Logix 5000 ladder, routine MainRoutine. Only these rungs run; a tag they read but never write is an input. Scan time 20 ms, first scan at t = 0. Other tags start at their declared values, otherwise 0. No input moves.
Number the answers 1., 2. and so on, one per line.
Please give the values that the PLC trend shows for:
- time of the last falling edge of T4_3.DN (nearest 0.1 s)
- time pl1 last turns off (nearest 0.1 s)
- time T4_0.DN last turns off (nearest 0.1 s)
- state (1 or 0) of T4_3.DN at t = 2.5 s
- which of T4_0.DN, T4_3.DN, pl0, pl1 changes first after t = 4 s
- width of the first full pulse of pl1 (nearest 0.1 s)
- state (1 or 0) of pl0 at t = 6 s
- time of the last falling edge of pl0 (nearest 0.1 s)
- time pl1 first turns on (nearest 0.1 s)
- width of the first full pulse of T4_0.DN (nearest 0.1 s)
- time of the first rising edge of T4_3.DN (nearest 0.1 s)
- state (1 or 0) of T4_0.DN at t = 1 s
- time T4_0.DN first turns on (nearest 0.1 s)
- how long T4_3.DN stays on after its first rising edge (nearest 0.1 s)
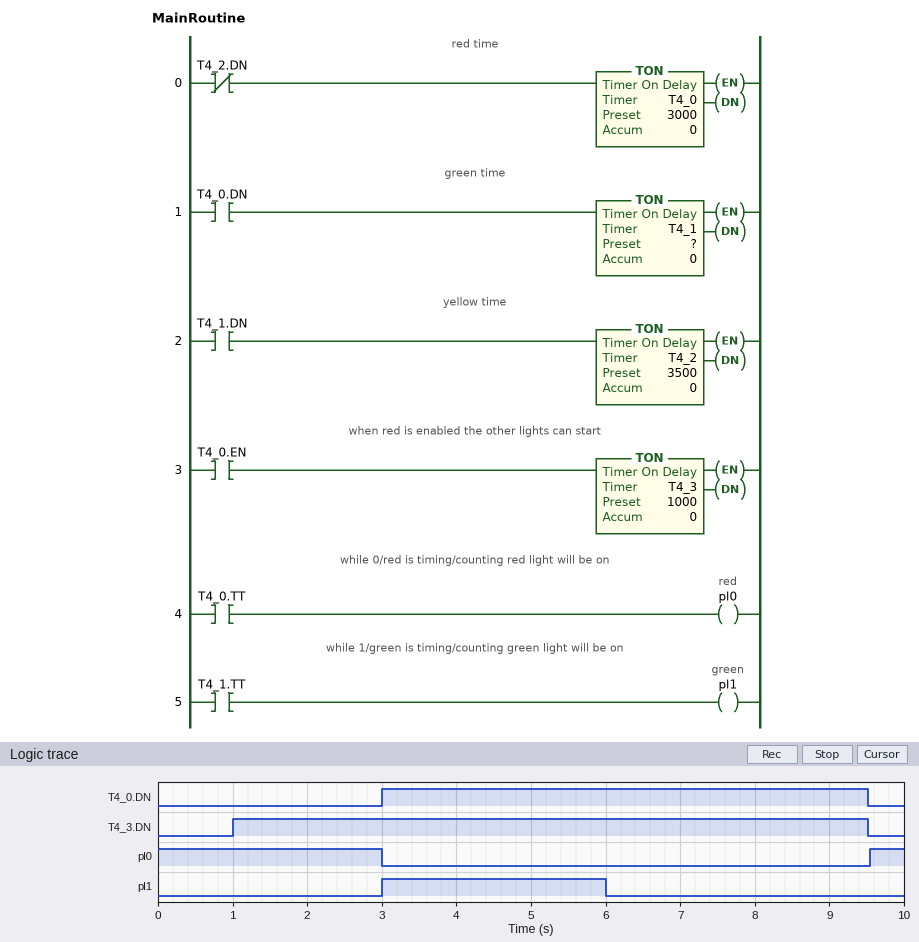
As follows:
1. 9.5 s
2. 6.0 s
3. 9.5 s
4. 1
5. pl1
6. 3.0 s
7. 0
8. 3.0 s
9. 3.0 s
10. 6.5 s
11. 1.0 s
12. 0
13. 3.0 s
14. 8.5 s
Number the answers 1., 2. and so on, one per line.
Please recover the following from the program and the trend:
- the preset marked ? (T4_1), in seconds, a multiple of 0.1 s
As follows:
1. 3.0 s
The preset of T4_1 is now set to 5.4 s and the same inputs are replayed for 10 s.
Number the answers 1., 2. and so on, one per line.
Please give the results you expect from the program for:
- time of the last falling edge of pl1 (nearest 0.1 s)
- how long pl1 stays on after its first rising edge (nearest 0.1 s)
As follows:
1. 8.4 s
2. 5.4 s
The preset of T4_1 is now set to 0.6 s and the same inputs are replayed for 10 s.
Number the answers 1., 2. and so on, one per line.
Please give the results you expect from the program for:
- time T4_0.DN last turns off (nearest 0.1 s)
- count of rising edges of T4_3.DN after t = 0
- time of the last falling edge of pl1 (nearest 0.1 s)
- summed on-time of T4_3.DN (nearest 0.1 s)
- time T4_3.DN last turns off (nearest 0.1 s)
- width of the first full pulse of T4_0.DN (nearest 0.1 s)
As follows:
1. 7.1 s
2. 2
3. 3.6 s
4. 8.0 s
5. 7.1 s
6. 4.1 s
